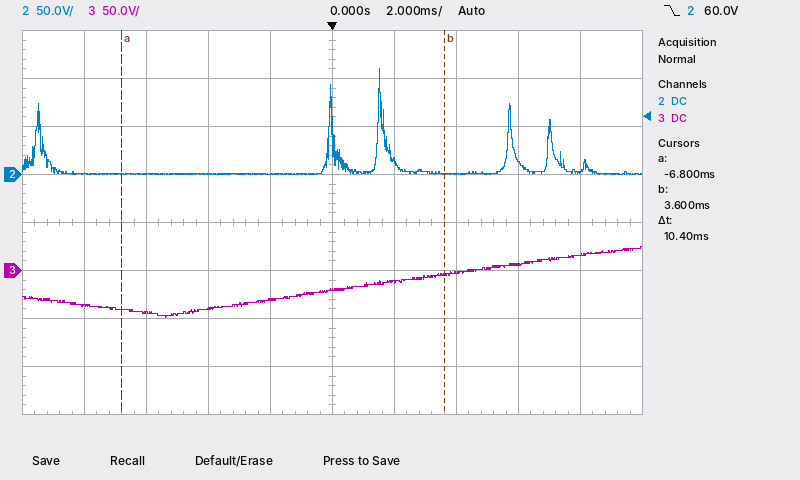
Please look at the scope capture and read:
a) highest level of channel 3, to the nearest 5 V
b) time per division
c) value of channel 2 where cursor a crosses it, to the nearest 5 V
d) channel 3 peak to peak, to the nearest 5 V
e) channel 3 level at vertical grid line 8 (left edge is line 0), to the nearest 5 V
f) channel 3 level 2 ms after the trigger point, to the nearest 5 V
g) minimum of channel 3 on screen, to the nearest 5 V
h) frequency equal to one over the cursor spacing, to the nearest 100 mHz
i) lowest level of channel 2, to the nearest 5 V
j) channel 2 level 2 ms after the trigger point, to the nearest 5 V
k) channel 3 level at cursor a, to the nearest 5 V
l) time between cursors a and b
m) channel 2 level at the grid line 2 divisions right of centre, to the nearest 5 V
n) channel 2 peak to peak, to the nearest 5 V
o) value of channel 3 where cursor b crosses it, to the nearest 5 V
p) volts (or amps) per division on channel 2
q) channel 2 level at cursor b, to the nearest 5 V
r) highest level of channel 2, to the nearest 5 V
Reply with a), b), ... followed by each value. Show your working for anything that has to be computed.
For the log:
a) 25 V
b) 2 ms
c) 0 V
d) 25 V − (-50 V) = 75 V
e) 5 V
f) -10 V
g) -50 V
h) 1 / 10.4 ms ≈ 96.2 Hz
i) 0 V
j) 15 V
k) -40 V
l) 10.4 ms
m) 0 V
n) 110 V − (0 V) = 110 V
o) -5 V
p) 50 V
q) 0 V
r) 110 V
